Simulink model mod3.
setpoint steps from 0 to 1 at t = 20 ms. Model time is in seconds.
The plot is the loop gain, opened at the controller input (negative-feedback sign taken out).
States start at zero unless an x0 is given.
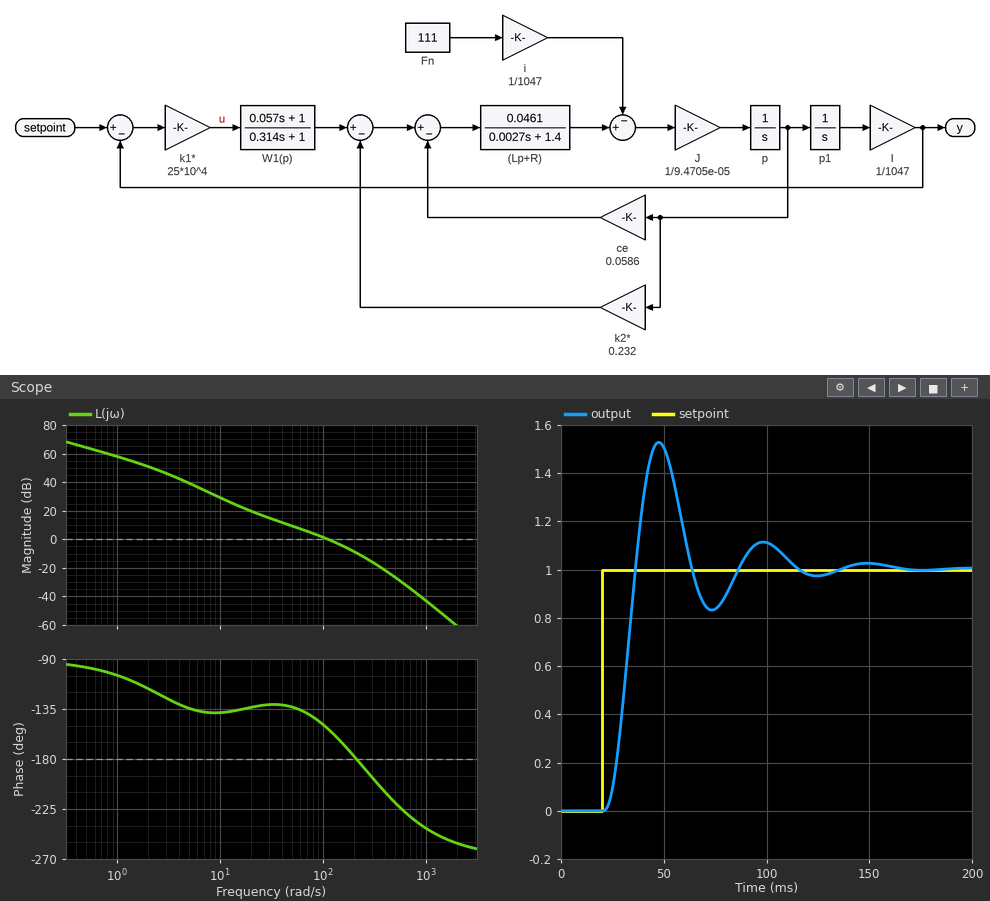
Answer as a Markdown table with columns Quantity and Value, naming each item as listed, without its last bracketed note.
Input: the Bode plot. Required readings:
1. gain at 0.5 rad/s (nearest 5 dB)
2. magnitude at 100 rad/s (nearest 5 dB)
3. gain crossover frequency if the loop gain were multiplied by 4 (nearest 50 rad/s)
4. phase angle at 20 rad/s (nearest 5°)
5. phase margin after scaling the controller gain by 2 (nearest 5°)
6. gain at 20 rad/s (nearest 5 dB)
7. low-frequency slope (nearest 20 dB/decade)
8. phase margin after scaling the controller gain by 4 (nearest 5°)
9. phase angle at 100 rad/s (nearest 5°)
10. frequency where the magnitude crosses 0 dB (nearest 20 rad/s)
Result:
| Quantity | Value |
|---|---|
| gain at 0.5 rad/s | 65 dB |
| magnitude at 100 rad/s | 0 dB |
| gain crossover frequency if the loop gain were multiplied by 4 | 250 rad/s |
| phase angle at 20 rad/s | -135° |
| phase margin after scaling the controller gain by 2 | 10° |
| gain at 20 rad/s | 20 dB |
| low-frequency slope | -20 dB/decade |
| phase margin after scaling the controller gain by 4 | -5° |
| phase angle at 100 rad/s | -150° |
| frequency where the magnitude crosses 0 dB | 120 rad/s |
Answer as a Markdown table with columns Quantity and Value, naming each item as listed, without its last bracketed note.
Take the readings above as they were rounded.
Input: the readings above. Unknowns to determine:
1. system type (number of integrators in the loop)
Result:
| Quantity | Value |
|---|---|
| system type | 1 |
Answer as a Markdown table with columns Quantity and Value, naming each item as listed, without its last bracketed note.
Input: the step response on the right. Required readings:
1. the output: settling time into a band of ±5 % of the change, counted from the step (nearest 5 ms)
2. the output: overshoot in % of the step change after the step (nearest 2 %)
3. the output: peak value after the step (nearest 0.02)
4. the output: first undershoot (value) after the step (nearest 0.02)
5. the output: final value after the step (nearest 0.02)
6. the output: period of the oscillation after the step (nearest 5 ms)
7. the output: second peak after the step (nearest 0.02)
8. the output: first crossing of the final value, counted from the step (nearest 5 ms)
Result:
| Quantity | Value |
|---|---|
| the output: settling time into a band of ±5 % of the change, counted from the step | 90 ms |
| the output: overshoot in % of the step change after the step | 52 % |
| the output: peak value after the step | 1.52 |
| the output: first undershoot (value) after the step | 0.84 |
| the output: final value after the step | 1.00 |
| the output: period of the oscillation after the step | 50 ms |
| the output: second peak after the step | 1.12 |
| the output: first crossing of the final value, counted from the step | 15 ms |
